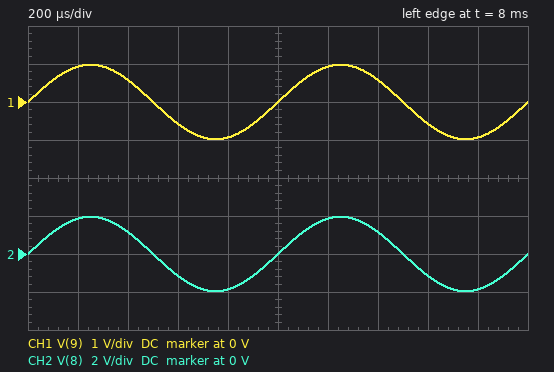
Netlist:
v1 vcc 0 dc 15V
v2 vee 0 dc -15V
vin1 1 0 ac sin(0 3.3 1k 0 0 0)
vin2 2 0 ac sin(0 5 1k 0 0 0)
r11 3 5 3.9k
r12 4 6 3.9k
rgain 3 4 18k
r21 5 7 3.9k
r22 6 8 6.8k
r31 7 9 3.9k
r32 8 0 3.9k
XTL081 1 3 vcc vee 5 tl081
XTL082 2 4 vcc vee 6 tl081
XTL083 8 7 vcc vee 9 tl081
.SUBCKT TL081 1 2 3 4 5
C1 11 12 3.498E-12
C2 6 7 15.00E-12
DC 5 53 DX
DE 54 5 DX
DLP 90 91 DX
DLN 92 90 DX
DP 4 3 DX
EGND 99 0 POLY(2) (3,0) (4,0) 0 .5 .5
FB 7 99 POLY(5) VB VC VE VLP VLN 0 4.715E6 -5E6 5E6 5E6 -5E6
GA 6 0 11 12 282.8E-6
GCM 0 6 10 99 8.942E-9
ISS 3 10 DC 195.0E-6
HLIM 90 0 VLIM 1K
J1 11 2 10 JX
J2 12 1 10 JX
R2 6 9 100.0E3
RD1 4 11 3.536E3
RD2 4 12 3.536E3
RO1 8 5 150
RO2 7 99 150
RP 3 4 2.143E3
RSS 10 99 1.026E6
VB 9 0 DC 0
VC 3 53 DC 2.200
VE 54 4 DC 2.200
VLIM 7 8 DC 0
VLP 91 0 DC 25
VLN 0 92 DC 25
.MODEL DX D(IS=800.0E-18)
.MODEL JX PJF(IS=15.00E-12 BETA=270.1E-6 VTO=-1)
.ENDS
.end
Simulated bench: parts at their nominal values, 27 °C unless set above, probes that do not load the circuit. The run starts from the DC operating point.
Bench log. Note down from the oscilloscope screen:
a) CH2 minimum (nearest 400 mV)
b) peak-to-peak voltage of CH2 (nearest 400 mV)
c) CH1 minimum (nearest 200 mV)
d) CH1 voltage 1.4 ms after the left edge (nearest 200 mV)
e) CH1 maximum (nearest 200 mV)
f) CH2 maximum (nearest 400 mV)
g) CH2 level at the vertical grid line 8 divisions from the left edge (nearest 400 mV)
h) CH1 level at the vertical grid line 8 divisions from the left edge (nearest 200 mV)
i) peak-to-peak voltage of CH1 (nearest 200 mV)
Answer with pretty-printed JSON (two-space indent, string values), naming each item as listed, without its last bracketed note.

{
  "CH2 minimum": "-2.0 V",
  "peak-to-peak voltage of CH2": "4.0 V",
  "CH1 minimum": "-1.0 V",
  "CH1 voltage 1.4 ms after the left edge": "600 mV",
  "CH1 maximum": "1.0 V",
  "CH2 maximum": "2.0 V",
  "CH2 level at the vertical grid line 8 divisions from the left edge": "-1.2 V",
  "CH1 level at the vertical grid line 8 divisions from the left edge": "-600 mV",
  "peak-to-peak voltage of CH1": "2.0 V"
}
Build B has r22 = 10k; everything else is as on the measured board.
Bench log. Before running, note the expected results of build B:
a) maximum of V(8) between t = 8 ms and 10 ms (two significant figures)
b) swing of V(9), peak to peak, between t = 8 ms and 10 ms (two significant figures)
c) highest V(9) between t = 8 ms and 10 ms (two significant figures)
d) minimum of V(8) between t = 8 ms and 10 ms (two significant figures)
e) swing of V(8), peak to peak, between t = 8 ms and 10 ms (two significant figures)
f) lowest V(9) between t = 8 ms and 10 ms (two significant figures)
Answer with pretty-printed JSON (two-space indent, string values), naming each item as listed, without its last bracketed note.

{
  "maximum of V(8) between t = 8 ms and 10 ms": "1.5 V",
  "swing of V(9), peak to peak, between t = 8 ms and 10 ms": "160 mV",
  "highest V(9) between t = 8 ms and 10 ms": "81 mV",
  "minimum of V(8) between t = 8 ms and 10 ms": "-1.5 V",
  "swing of V(8), peak to peak, between t = 8 ms and 10 ms": "3.0 V",
  "lowest V(9) between t = 8 ms and 10 ms": "-81 mV"
}
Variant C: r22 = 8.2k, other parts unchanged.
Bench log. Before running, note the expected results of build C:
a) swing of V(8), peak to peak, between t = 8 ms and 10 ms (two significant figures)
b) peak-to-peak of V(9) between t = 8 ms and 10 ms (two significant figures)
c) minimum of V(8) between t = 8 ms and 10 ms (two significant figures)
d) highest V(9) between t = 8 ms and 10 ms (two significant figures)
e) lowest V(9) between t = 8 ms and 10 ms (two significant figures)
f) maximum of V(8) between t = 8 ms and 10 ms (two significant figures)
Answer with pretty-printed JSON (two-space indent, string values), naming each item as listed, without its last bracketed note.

{
  "swing of V(8), peak to peak, between t = 8 ms and 10 ms": "3.5 V",
  "peak-to-peak of V(9) between t = 8 ms and 10 ms": "1.1 V",
  "minimum of V(8) between t = 8 ms and 10 ms": "-1.7 V",
  "highest V(9) between t = 8 ms and 10 ms": "530 mV",
  "lowest V(9) between t = 8 ms and 10 ms": "-530 mV",
  "maximum of V(8) between t = 8 ms and 10 ms": "1.7 V"
}
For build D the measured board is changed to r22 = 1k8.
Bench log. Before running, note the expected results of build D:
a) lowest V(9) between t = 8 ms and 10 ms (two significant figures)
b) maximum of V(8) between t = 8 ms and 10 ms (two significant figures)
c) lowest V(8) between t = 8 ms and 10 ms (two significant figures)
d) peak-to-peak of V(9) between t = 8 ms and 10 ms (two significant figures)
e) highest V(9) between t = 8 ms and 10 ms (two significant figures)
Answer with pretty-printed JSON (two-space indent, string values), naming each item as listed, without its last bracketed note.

{
  "lowest V(9) between t = 8 ms and 10 ms": "-4.4 V",
  "maximum of V(8) between t = 8 ms and 10 ms": "3.7 V",
  "lowest V(8) between t = 8 ms and 10 ms": "-3.7 V",
  "peak-to-peak of V(9) between t = 8 ms and 10 ms": "8.8 V",
  "highest V(9) between t = 8 ms and 10 ms": "4.4 V"
}
